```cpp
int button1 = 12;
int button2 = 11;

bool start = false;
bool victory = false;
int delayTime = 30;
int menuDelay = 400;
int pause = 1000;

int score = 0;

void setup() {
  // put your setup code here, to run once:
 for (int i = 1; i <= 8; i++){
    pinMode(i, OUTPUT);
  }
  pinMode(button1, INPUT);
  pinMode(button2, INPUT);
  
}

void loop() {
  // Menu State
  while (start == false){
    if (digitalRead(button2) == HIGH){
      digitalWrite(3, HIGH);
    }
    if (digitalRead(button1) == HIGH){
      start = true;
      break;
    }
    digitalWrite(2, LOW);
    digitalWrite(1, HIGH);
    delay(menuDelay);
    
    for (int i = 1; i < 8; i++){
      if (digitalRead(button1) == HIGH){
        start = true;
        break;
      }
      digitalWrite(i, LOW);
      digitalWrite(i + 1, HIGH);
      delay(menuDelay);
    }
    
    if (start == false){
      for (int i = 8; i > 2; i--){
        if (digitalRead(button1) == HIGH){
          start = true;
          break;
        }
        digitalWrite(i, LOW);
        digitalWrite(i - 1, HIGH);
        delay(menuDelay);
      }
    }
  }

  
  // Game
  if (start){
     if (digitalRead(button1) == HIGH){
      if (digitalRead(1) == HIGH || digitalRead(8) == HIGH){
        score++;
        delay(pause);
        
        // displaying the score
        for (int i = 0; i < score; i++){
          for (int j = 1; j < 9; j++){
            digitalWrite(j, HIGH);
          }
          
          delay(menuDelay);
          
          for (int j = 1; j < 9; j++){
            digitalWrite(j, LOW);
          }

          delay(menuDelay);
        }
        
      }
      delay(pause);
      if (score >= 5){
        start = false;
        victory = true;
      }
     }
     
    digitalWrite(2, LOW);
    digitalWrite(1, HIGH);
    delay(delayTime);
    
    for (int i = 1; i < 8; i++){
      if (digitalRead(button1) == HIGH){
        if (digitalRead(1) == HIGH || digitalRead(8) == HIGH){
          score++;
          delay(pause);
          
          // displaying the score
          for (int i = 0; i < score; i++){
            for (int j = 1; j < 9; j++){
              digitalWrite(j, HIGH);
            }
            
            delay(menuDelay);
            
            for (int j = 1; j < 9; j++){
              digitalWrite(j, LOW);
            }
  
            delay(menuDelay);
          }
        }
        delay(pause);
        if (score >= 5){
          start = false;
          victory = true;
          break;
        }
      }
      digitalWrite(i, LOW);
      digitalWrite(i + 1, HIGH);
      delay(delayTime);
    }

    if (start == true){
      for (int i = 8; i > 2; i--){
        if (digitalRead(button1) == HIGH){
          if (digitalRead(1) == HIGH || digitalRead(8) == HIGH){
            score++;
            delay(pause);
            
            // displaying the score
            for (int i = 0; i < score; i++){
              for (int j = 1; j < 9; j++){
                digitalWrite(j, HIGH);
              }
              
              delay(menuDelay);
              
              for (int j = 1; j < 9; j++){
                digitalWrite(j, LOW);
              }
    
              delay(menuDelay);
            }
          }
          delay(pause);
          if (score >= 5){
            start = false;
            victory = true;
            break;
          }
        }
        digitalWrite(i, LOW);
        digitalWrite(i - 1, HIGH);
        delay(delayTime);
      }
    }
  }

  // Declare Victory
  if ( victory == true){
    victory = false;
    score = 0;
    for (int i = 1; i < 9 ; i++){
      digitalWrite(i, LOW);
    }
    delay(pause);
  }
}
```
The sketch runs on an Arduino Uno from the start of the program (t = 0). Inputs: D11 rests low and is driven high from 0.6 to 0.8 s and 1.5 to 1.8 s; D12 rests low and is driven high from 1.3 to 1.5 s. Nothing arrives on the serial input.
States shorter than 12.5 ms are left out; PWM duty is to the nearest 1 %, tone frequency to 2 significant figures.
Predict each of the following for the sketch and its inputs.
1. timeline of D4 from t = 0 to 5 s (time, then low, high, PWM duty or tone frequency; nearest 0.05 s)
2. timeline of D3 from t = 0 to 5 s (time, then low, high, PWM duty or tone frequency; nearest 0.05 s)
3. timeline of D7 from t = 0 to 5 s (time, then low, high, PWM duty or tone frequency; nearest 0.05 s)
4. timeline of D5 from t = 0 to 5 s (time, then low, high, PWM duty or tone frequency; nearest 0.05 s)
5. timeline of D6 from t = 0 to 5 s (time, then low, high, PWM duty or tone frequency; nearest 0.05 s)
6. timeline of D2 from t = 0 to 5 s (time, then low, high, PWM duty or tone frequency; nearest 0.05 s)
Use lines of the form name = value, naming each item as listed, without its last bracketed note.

timeline of D4 from t = 0 to 5 s = 0 s low; 1.2 s high; 1.6 s low; 4.4 s high; 4.8 s low
timeline of D3 from t = 0 to 5 s = 0 s low; 0.8 s high; 1.2 s low; 4.8 s high
timeline of D7 from t = 0 to 5 s = 0 s low; 2.4 s high; 2.8 s low; 3.2 s high; 3.6 s low
timeline of D5 from t = 0 to 5 s = 0 s low; 1.6 s high; 2 s low; 4 s high; 4.4 s low
timeline of D6 from t = 0 to 5 s = 0 s low; 2 s high; 2.4 s low; 3.6 s high; 4 s low
timeline of D2 from t = 0 to 5 s = 0 s low; 0.4 s high; 0.8 s low
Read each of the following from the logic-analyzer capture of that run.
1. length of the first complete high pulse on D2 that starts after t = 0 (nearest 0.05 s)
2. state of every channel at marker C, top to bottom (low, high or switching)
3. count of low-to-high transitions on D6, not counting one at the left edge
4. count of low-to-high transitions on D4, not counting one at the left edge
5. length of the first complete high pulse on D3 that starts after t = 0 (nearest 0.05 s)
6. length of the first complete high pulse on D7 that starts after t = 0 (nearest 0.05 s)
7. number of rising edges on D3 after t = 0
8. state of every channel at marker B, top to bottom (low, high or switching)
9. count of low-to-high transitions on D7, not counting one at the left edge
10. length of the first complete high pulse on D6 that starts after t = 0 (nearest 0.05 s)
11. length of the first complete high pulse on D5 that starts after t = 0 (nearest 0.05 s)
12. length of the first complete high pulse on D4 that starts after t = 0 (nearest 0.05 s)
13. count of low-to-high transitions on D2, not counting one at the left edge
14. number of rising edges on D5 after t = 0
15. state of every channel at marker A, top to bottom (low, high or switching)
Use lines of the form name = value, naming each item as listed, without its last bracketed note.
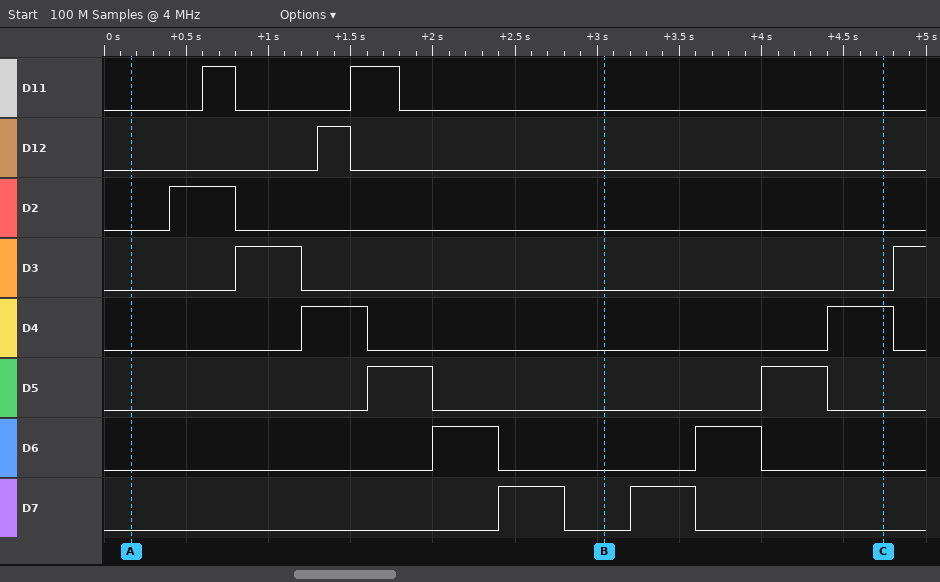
length of the first complete high pulse on D2 that starts after t = 0 = 0.40 s
state of every channel at marker C, top to bottom = D11 low, D12 low, D2 low, D3 low, D4 high, D5 low, D6 low, D7 low
count of low-to-high transitions on D6, not counting one at the left edge = 2
count of low-to-high transitions on D4, not counting one at the left edge = 2
length of the first complete high pulse on D3 that starts after t = 0 = 0.40 s
length of the first complete high pulse on D7 that starts after t = 0 = 0.40 s
number of rising edges on D3 after t = 0 = 2
state of every channel at marker B, top to bottom = D11 low, D12 low, D2 low, D3 low, D4 low, D5 low, D6 low, D7 low
count of low-to-high transitions on D7, not counting one at the left edge = 2
length of the first complete high pulse on D6 that starts after t = 0 = 0.40 s
length of the first complete high pulse on D5 that starts after t = 0 = 0.40 s
length of the first complete high pulse on D4 that starts after t = 0 = 0.40 s
count of low-to-high transitions on D2, not counting one at the left edge = 1
number of rising edges on D5 after t = 0 = 2
state of every channel at marker A, top to bottom = D11 low, D12 low, D2 low, D3 low, D4 low, D5 low, D6 low, D7 low
